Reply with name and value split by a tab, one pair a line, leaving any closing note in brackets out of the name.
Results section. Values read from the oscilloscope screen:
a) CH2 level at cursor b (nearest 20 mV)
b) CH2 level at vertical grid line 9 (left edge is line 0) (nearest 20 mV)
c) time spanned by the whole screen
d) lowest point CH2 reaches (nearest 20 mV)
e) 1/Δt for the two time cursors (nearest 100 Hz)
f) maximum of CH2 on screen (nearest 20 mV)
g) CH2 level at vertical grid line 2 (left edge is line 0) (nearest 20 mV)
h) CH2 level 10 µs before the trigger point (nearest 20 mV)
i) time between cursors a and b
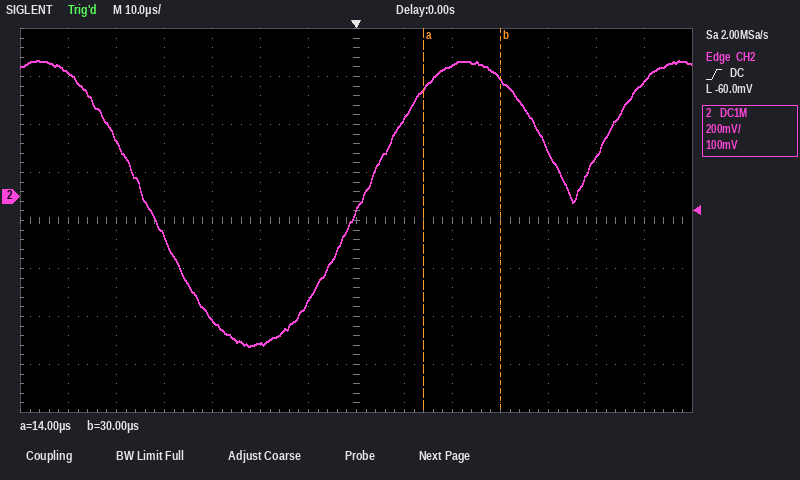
CH2 level at cursor b	480 mV
CH2 level at vertical grid line 9 (left edge is line 0)	540 mV
time spanned by the whole screen	140 µs
lowest point CH2 reaches	-620 mV
1/Δt for the two time cursors	62.5 kHz
maximum of CH2 on screen	560 mV
CH2 level at vertical grid line 2 (left edge is line 0)	240 mV
CH2 level 10 µs before the trigger point	-440 mV
time between cursors a and b	16 µs
